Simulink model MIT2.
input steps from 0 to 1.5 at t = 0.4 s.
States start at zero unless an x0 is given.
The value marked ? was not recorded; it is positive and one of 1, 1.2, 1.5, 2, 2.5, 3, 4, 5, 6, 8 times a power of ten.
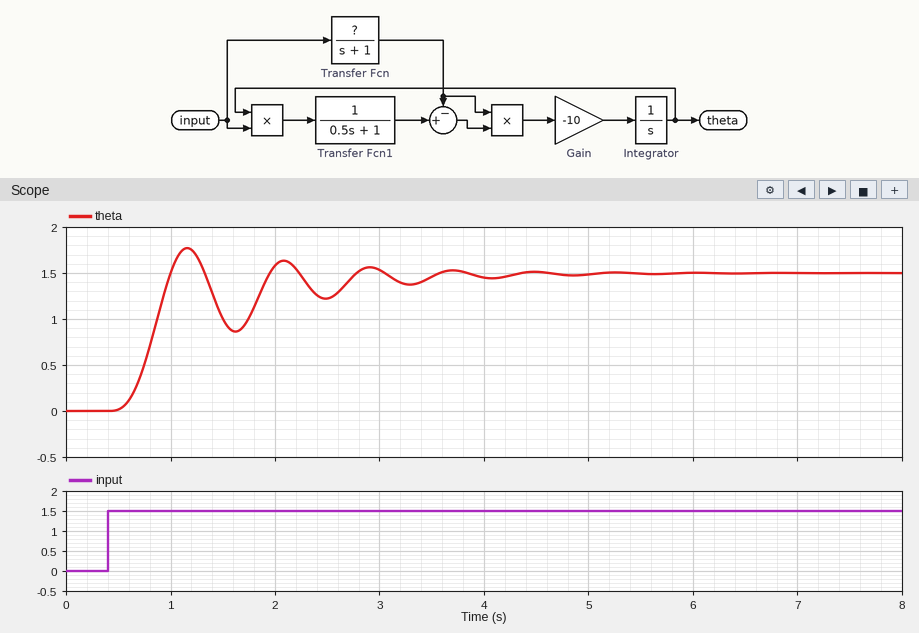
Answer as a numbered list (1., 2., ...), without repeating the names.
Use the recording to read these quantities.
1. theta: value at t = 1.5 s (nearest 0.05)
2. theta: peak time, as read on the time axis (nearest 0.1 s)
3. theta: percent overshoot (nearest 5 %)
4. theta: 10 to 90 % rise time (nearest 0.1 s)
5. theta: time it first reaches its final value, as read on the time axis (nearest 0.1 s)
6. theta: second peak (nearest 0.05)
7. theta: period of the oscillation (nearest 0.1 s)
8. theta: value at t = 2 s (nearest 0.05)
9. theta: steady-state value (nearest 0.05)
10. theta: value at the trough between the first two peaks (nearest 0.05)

1. 1.00
2. 1.2 s
3. 20 %
4. 0.3 s
5. 1.0 s
6. 1.65
7. 0.9 s
8. 1.60
9. 1.50
10. 0.85
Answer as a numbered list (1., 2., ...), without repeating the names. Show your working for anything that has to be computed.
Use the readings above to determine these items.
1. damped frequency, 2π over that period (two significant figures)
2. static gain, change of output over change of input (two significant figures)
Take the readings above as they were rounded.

1. 2π / 0.9 = 7.0 rad/s
2. (1.5 - 0) / (1.5 - 0) = 1.0
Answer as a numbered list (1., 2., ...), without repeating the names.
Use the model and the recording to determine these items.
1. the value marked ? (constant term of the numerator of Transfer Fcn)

1. 1.5
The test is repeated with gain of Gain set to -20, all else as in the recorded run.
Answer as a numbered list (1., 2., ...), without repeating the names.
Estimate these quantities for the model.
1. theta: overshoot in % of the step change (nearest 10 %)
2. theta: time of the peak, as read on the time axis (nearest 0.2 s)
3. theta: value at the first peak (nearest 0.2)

1. 20 %
2. 1.0 s
3. 1.8
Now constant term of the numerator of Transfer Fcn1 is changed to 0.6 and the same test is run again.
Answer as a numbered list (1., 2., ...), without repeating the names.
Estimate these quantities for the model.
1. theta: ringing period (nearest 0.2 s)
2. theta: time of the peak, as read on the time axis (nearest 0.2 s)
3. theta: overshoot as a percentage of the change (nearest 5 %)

1. 1.2 s
2. 1.4 s
3. 15 %
